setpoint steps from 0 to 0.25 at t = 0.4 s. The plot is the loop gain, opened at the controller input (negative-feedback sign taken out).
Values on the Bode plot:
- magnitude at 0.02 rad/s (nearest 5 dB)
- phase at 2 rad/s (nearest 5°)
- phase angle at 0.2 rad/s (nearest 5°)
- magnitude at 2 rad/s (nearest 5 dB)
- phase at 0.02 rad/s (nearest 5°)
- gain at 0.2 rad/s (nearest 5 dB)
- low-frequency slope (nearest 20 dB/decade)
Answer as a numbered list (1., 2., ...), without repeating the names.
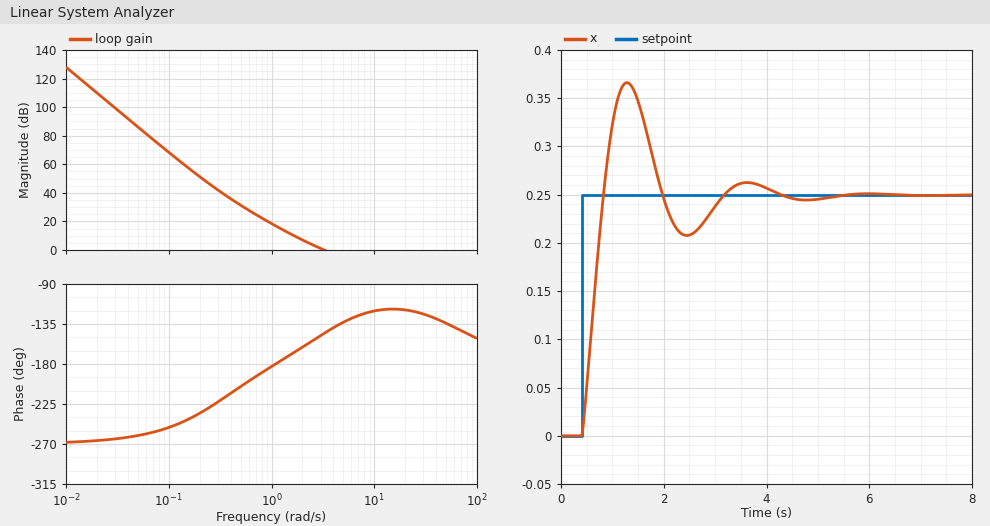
1. 110 dB
2. -160°
3. -235°
4. 5 dB
5. -265°
6. 50 dB
7. -60 dB/decade
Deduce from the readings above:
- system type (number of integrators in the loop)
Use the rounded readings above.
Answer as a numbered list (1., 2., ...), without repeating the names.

1. 3
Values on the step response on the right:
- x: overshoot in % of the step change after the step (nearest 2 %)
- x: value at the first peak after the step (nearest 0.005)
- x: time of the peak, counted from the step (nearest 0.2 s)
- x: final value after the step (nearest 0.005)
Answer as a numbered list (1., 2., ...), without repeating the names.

1. 46 %
2. 0.365
3. 0.8 s
4. 0.250
